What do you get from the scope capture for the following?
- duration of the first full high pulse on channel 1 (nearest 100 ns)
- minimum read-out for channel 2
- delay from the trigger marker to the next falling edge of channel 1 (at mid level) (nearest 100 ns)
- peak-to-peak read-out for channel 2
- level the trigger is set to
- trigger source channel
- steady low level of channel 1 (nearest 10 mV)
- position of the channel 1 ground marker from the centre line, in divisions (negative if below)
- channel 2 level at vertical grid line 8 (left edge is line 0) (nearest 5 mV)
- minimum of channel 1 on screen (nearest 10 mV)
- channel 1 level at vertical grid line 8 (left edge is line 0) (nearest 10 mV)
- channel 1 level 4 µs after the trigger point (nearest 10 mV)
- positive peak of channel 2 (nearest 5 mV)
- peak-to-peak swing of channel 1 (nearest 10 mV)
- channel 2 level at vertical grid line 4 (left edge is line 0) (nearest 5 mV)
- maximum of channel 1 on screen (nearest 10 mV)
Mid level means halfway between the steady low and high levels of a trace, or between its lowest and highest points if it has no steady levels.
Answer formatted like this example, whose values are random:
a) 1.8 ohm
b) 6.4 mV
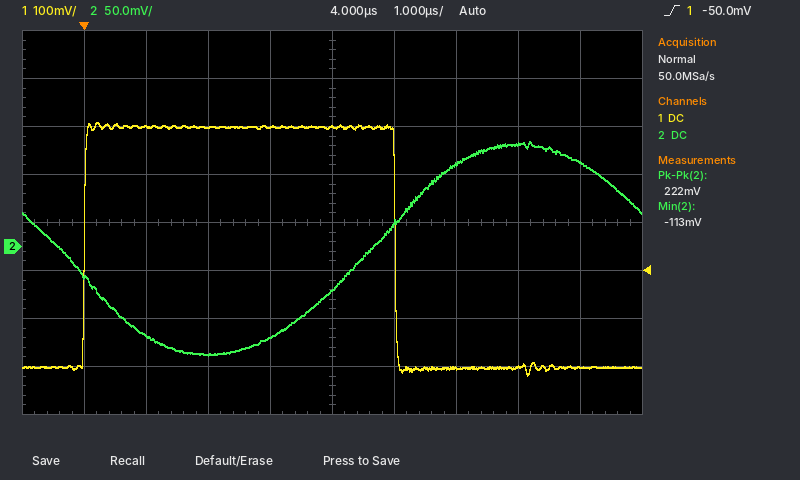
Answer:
a) 5.0 µs
b) -113 mV
c) 5.0 µs
d) 222 mV
e) -50.0 mV
f) channel 1
g) -250 mV
h) -0.5 div
i) 105 mV
j) -270 mV
k) -250 mV
l) 250 mV
m) 110 mV
n) 530 mV
o) -95 mV
p) 260 mV
